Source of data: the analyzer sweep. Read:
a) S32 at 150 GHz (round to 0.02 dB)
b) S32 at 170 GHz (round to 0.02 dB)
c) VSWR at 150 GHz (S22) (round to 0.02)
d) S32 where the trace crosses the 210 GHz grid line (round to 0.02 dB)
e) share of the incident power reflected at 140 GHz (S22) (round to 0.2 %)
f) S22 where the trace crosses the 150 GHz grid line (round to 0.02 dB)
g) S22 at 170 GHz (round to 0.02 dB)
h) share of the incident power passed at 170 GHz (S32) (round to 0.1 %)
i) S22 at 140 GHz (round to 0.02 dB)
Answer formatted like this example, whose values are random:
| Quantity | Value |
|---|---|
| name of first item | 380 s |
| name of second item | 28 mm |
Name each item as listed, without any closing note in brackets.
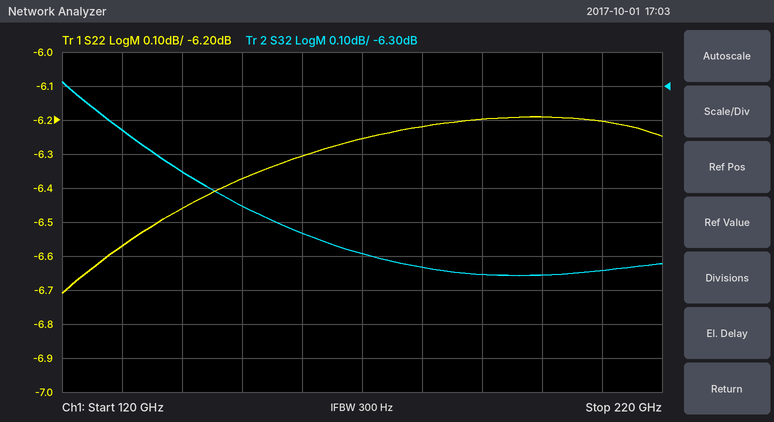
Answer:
| Quantity | Value |
|---|---|
| S32 at 150 GHz | -6.66 dB |
| S32 at 170 GHz | -6.80 dB |
| VSWR at 150 GHz (S22) | 2.84 |
| S32 where the trace crosses the 210 GHz grid line | -6.84 dB |
| share of the incident power reflected at 140 GHz (S22) | 22.6 % |
| S22 where the trace crosses the 150 GHz grid line | -6.38 dB |
| S22 at 170 GHz | -6.26 dB |
| share of the incident power passed at 170 GHz (S32) | 20.9 % |
| S22 at 140 GHz | -6.46 dB |
